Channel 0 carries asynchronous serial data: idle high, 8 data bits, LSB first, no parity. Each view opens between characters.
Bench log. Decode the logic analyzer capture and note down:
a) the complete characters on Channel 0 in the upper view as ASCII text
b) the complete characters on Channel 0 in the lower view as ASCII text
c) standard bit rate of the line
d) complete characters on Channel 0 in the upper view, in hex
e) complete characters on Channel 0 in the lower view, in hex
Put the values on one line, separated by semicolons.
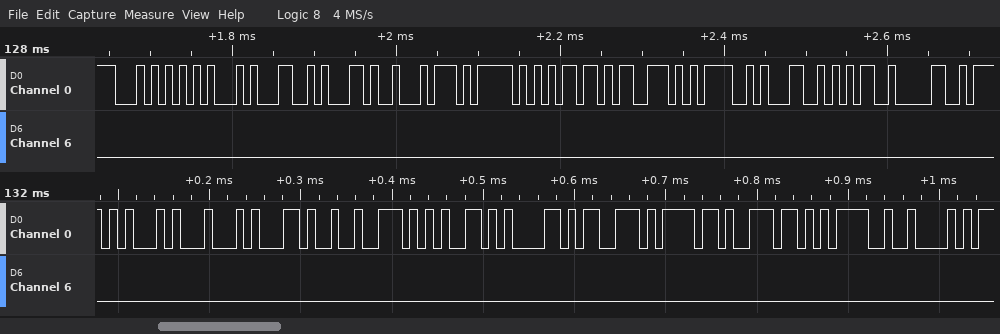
"TEL,t_ms=150"; "ED,reason=B"; 115200 baud; 54, 45, 4C, 2C, 74, 5F, 6D, 73, 3D, 31, 35, 30; 45, 44, 2C, 72, 65, 61, 73, 6F, 6E, 3D, 42
